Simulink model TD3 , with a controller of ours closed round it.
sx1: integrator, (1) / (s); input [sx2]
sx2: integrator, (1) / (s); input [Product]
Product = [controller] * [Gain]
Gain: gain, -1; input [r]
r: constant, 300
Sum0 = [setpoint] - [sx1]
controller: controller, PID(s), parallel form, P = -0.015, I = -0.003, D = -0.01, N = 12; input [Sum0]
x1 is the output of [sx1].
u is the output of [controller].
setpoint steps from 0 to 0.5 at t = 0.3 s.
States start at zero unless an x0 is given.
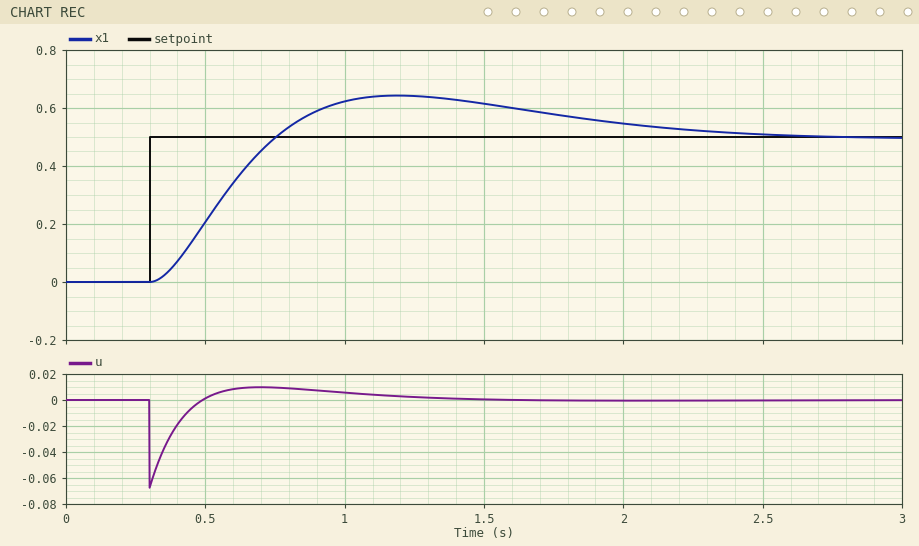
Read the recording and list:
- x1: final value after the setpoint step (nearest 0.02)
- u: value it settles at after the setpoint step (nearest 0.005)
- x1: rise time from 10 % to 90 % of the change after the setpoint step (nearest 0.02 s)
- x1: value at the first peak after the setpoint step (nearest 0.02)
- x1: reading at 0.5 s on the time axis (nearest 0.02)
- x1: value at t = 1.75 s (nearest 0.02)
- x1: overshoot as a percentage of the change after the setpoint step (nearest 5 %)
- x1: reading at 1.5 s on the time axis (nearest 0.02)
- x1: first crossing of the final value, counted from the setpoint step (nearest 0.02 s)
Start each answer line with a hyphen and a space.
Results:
- 0.50
- 0.000
- 0.32 s
- 0.64
- 0.20
- 0.58
- 30 %
- 0.62
- 0.46 s
